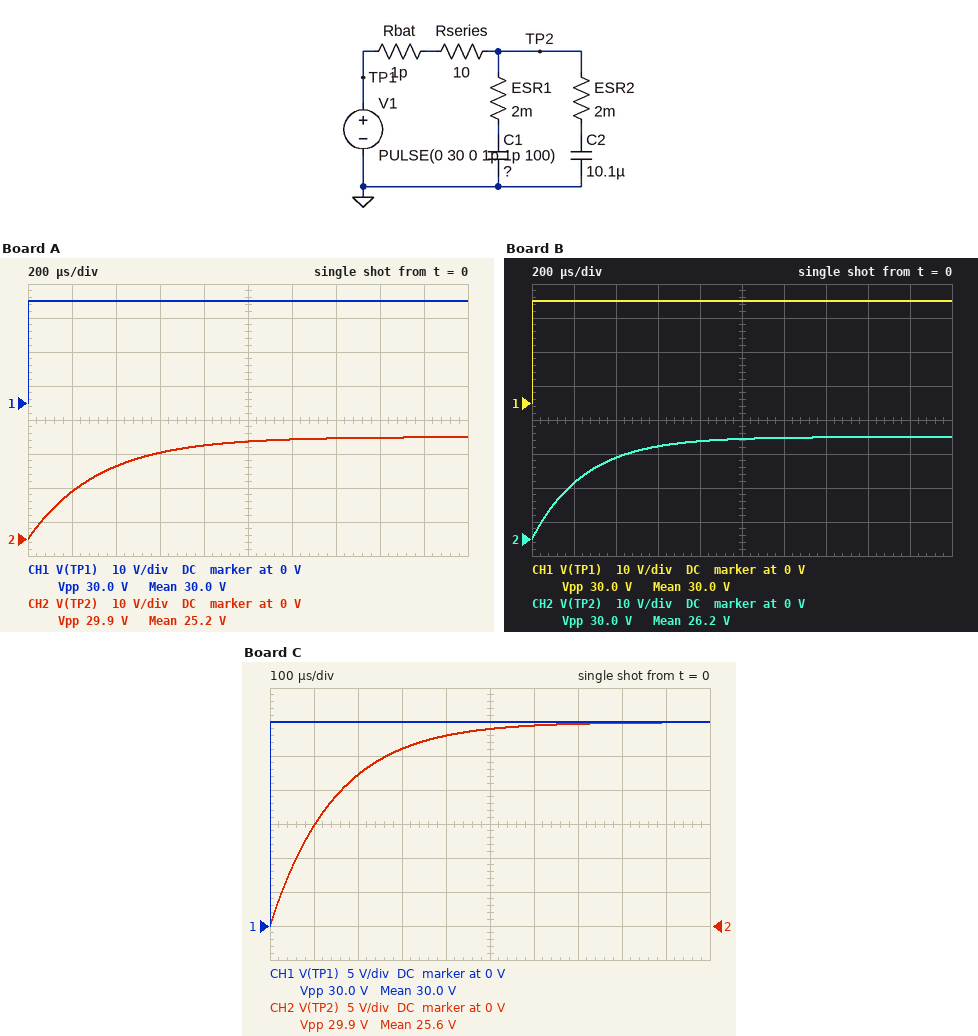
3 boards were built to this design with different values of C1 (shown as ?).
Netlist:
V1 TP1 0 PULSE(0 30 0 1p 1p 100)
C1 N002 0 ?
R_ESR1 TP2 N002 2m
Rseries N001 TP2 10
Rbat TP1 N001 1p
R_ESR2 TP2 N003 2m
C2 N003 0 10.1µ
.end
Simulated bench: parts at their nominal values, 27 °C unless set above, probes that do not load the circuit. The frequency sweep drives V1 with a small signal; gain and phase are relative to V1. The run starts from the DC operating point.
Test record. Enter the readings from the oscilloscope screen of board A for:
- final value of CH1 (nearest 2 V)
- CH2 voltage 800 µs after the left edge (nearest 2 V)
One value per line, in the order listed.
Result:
30 V
28 V
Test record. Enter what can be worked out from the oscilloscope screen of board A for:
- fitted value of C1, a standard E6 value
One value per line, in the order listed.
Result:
22 µF
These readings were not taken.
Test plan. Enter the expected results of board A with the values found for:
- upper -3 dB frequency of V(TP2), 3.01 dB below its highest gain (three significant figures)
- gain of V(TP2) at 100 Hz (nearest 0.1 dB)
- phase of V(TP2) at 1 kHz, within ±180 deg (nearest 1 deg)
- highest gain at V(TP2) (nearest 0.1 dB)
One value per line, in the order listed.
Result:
496 Hz
-0.2 dB
-64 deg
0 dB
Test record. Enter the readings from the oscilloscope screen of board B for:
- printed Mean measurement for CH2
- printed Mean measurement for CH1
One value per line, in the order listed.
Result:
26.2 V
30.0 V
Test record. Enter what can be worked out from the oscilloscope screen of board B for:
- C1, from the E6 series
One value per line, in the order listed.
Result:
15 µF
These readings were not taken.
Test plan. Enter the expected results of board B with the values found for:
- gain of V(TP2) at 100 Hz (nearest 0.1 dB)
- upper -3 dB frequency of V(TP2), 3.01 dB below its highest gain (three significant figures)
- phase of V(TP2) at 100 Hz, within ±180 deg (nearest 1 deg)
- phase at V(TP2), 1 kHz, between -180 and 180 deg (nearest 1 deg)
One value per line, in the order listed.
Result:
-0.1 dB
634 Hz
-9 deg
-58 deg
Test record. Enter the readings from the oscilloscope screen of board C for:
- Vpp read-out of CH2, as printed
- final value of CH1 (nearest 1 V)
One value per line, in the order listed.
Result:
29.9 V
30 V
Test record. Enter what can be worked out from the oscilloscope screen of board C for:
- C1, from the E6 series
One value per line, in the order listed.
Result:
4.7 µF
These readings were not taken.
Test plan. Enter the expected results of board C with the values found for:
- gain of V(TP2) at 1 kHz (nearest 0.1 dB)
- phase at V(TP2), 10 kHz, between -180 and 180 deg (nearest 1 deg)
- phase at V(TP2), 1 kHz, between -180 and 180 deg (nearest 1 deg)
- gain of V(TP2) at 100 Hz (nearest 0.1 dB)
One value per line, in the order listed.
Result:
-2.7 dB
-84 deg
-43 deg
0 dB
